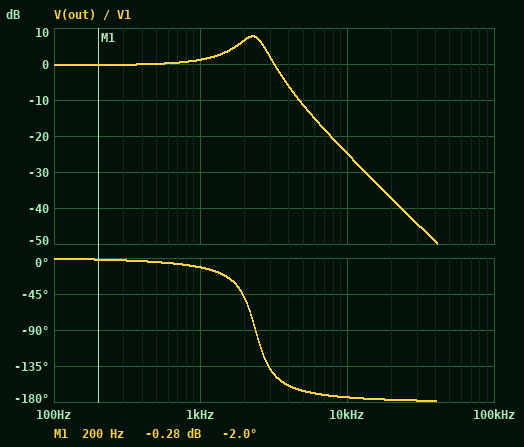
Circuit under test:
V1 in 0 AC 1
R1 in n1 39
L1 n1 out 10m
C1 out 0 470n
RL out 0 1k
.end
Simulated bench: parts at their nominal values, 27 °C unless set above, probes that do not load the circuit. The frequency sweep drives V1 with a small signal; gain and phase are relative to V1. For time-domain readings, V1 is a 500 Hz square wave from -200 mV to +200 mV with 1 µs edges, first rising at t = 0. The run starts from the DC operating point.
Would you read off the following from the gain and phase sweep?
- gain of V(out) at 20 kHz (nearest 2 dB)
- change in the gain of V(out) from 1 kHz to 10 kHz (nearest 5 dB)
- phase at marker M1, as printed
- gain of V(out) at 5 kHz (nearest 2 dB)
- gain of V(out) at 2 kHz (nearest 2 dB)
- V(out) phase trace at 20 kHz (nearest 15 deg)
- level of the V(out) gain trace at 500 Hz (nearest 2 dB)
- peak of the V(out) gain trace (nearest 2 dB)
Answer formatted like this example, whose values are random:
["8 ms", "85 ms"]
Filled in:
["-38 dB", "-25 dB", "-2.0 deg", "-12 dB", "6 dB", "-180 deg", "0 dB", "8 dB"]
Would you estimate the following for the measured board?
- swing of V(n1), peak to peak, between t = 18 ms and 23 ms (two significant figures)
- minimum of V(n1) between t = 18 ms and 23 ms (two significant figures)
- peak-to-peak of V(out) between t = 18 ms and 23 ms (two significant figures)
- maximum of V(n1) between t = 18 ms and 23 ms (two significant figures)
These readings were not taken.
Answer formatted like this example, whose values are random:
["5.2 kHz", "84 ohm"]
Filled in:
["460 mV", "-230 mV", "790 mV", "230 mV"]
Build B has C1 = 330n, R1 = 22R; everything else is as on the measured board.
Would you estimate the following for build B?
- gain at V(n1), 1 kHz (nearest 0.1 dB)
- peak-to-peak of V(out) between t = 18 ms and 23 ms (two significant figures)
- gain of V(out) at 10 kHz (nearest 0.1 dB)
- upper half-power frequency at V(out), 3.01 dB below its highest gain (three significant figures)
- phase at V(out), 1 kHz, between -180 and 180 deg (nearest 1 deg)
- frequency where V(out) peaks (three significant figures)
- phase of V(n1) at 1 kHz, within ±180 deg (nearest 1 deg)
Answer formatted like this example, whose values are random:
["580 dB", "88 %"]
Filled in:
["-0.3 dB", "880 mV", "-21.6 dB", "3.13 kHz", "-7 deg", "2.74 kHz", "-3 deg"]
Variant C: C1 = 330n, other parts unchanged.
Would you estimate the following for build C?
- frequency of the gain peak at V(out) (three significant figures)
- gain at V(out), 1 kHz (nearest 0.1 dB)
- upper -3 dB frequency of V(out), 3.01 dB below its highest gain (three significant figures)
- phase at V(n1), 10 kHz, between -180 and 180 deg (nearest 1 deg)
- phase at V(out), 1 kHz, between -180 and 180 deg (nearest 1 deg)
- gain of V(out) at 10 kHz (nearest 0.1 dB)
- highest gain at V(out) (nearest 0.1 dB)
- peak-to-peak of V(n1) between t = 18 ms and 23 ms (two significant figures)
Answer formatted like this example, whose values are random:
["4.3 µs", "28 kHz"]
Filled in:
["2.71 kHz", "0.7 dB", "3.23 kHz", "4 deg", "-9 deg", "-21.6 dB", "8.0 dB", "450 mV"]
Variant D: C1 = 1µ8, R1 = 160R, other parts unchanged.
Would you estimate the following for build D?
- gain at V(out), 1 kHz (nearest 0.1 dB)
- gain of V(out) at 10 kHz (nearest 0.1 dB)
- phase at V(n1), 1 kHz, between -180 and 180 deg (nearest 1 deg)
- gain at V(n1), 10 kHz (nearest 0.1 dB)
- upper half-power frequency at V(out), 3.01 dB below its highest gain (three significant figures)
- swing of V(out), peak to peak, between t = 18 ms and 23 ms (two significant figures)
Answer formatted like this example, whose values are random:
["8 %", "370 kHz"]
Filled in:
["-5.7 dB", "-37.2 dB", "-64 deg", "-0.3 dB", "787 Hz", "340 mV"]
